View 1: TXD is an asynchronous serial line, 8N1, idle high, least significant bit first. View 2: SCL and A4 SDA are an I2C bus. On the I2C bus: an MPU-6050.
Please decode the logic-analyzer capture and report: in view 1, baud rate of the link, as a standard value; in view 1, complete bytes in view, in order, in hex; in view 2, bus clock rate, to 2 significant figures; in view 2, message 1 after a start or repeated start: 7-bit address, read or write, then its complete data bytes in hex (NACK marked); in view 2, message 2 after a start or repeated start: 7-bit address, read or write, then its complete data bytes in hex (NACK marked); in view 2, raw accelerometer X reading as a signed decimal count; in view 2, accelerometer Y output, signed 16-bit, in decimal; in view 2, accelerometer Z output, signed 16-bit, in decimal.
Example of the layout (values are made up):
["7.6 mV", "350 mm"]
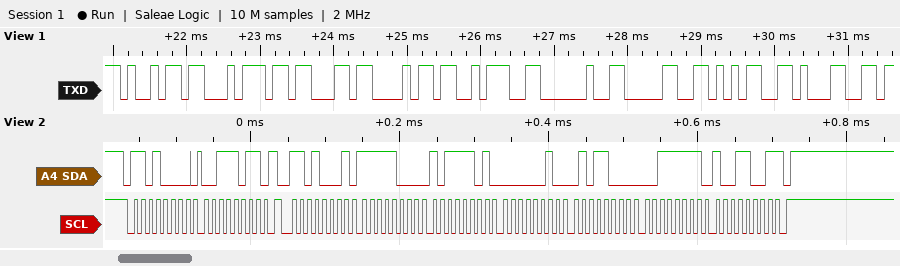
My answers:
["9600 baud", "69 74 63 68 3A 20 30 35 31", "100 kHz", "0x68 write: 3B", "0x68 read: F8 BD 02 58 3F 99 NACK", "-1859", "600", "16281"]
